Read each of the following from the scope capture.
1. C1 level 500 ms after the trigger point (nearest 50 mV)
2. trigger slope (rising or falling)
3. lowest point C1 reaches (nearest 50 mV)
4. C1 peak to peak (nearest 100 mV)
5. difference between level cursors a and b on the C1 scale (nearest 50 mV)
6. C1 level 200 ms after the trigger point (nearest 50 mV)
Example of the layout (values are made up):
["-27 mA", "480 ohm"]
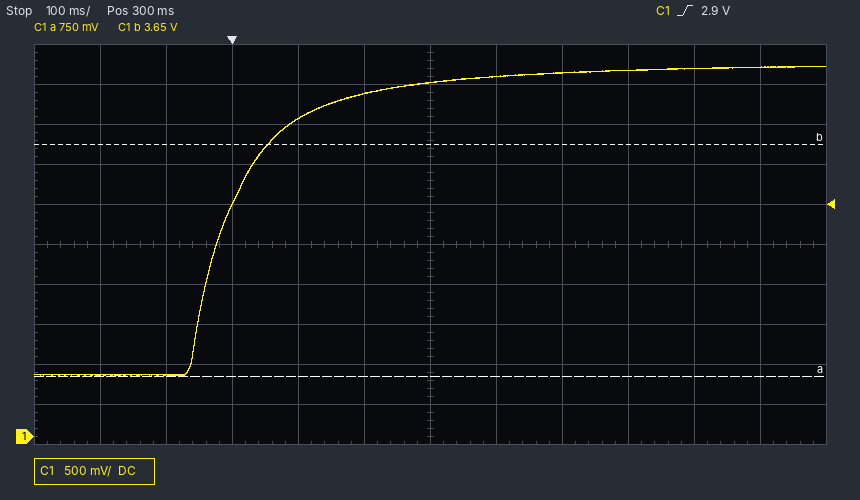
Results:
["4.55 V", "rising", "750 mV", "3.90 V", "2.90 V", "4.30 V"]
